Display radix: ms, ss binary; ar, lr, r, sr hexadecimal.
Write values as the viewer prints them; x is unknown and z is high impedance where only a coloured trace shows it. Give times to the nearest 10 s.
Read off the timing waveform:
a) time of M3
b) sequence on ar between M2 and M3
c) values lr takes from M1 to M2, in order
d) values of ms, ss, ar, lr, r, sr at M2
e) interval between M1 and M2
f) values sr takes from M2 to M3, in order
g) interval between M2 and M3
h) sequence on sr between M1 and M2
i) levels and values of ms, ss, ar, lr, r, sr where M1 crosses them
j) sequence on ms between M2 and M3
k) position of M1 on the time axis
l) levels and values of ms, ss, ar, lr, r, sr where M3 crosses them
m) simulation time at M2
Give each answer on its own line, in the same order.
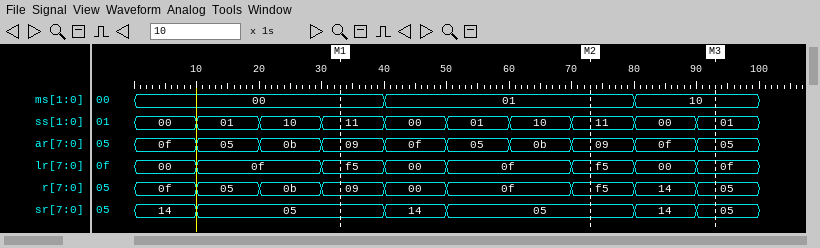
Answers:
90 s
09, 0f, 05
f5, 00, 0f, f5
ms=01, ss=11, ar=09, lr=f5, r=f5, sr=05
40 s
05, 14, 05
20 s
05, 14, 05
ms=00, ss=11, ar=09, lr=f5, r=09, sr=05
01, 10
30 s
ms=10, ss=01, ar=05, lr=0f, r=05, sr=05
70 s
